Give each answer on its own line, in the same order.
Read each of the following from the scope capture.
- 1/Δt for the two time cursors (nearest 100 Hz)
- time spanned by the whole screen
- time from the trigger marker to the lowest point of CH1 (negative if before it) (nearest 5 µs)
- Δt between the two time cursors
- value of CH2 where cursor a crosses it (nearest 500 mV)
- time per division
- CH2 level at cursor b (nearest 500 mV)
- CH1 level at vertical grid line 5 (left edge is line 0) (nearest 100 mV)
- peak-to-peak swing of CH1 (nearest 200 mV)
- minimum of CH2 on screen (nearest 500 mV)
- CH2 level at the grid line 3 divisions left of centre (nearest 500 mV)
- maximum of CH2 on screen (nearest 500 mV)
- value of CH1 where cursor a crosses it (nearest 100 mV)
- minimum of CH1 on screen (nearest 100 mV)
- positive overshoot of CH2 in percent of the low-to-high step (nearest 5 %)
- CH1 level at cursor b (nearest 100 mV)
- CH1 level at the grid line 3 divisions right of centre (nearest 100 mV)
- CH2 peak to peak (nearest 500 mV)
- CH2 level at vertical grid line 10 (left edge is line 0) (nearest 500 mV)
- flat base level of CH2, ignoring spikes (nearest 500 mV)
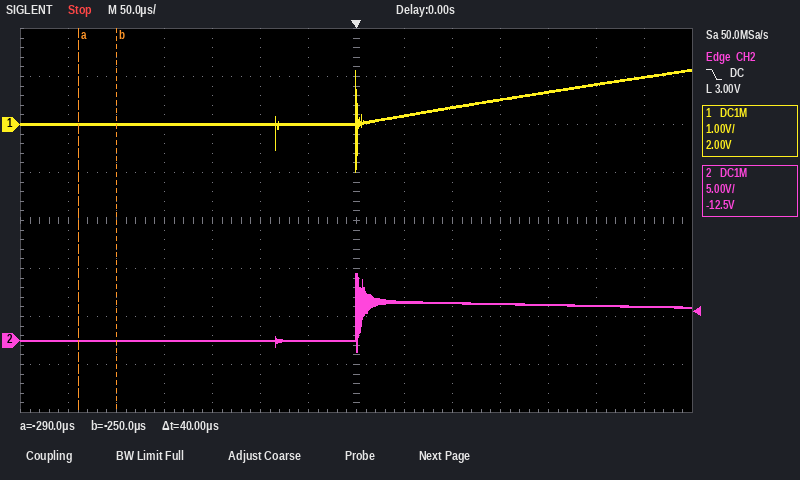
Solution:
25.0 kHz
700 µs
0 µs
40 µs
0.0 V
50 µs
0.0 V
0.0 V
2.2 V
-1.0 V
0.0 V
7.0 V
0.0 V
-1.0 V
85 %
0.0 V
500 mV
8.0 V
4.0 V
0.0 V
